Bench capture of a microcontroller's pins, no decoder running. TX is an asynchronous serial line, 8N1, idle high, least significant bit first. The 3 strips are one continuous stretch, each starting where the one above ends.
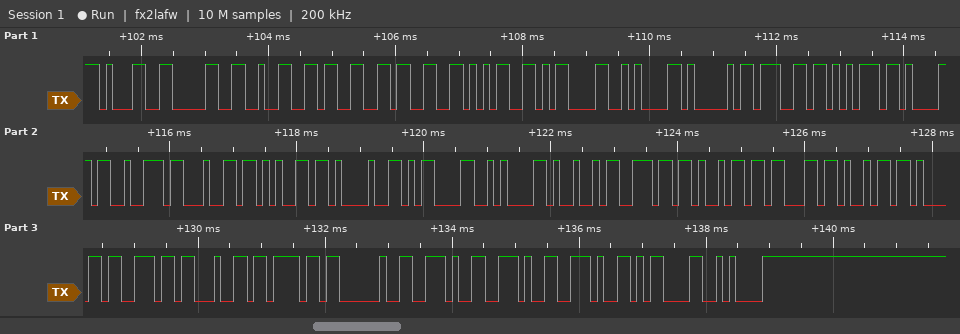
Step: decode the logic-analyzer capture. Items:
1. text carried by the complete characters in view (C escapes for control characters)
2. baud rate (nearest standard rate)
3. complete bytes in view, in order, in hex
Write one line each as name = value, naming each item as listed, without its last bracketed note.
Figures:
text carried by the complete characters in view = "102335\r\nAguarde!\r\nIniciando ...\r\n"
baud rate = 9600 baud
complete bytes in view, in order, in hex = 0x31 0x30 0x32 0x33 0x33 0x35 0x0D 0x0A 0x41 0x67 0x75 0x61 0x72 0x64 0x65 0x21 0x0D 0x0A 0x49 0x6E 0x69 0x63 0x69 0x61 0x6E 0x64 0x6F 0x20 0x2E 0x2E 0x2E 0x0D 0x0A
